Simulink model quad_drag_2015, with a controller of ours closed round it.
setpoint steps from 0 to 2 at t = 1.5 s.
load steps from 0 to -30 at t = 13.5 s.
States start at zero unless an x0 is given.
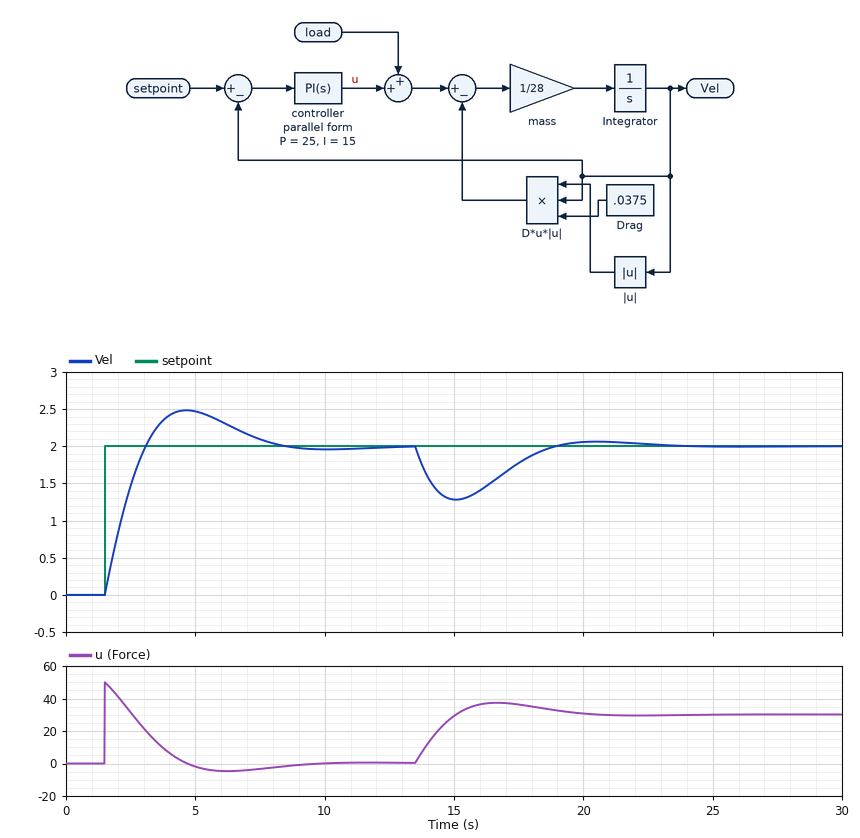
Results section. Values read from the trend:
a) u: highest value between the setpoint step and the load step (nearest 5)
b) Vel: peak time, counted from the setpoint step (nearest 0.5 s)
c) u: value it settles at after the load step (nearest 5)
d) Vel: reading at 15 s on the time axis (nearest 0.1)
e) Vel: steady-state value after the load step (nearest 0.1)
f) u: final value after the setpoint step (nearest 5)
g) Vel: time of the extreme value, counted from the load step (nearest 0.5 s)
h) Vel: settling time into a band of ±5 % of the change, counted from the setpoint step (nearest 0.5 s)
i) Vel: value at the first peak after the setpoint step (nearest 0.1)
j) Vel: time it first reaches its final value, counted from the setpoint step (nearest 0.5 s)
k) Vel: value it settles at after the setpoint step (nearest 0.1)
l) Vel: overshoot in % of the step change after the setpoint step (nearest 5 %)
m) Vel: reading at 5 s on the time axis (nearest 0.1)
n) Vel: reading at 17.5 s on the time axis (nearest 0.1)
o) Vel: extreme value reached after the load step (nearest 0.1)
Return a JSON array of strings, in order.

["50", "3.0 s", "30", "1.3", "2.0", "0", "1.5 s", "6.0 s", "2.5", "1.5 s", "2.0", "25 %", "2.5", "1.8", "1.3"]
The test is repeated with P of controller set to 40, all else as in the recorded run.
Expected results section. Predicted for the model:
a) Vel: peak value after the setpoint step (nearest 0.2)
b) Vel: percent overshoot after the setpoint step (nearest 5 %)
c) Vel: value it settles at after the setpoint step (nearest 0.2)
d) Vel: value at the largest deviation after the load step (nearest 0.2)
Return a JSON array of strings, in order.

["2.2", "15 %", "2.0", "1.4"]
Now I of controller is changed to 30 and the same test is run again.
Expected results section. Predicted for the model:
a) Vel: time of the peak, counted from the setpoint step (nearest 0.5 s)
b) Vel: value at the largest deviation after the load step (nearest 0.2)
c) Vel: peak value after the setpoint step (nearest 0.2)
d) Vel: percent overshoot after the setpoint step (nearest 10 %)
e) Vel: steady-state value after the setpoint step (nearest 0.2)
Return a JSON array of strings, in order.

["2.5 s", "1.4", "2.6", "30 %", "2.0"]
